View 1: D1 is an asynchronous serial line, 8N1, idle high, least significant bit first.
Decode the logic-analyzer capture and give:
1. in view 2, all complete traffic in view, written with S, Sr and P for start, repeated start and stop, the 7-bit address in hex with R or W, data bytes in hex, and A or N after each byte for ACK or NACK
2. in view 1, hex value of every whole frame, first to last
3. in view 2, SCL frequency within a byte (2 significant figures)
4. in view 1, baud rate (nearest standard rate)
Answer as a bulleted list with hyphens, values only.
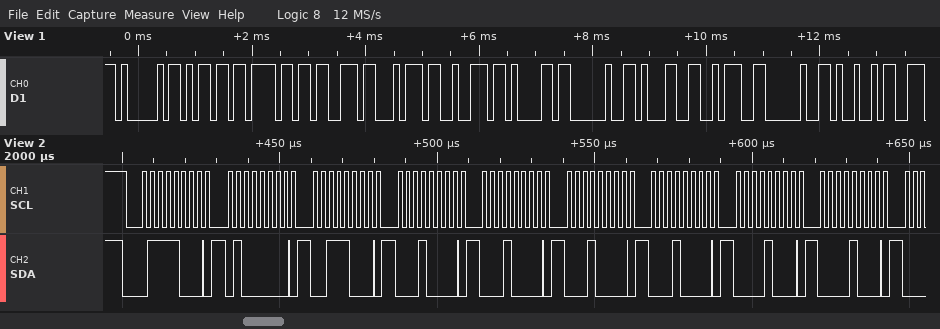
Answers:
- S 3CW A 40 A 38 A 10 A 10 A 10 A 10 A 08 A 08 A
- 41 6D 6F 73 74 72 61 20 31 3A 20 49
- 400 kHz
- 9600 baud
